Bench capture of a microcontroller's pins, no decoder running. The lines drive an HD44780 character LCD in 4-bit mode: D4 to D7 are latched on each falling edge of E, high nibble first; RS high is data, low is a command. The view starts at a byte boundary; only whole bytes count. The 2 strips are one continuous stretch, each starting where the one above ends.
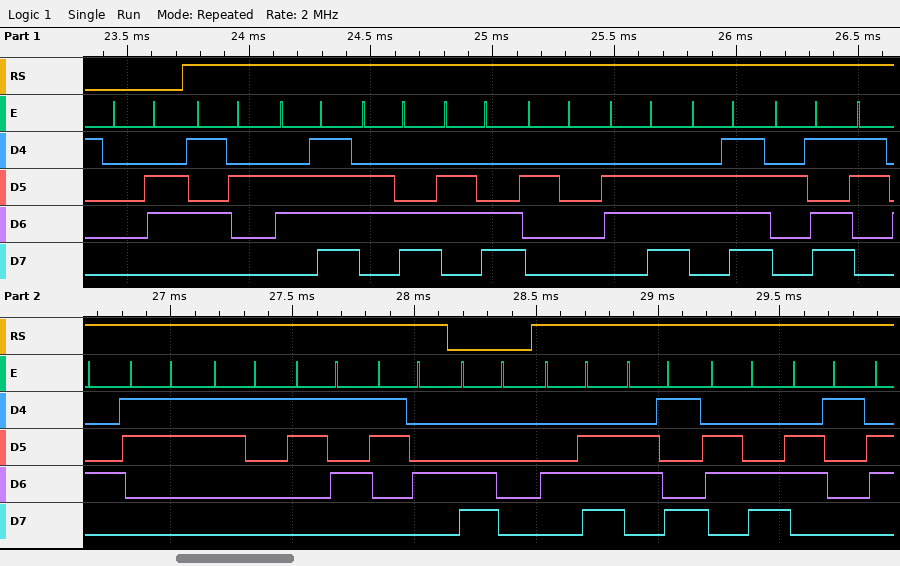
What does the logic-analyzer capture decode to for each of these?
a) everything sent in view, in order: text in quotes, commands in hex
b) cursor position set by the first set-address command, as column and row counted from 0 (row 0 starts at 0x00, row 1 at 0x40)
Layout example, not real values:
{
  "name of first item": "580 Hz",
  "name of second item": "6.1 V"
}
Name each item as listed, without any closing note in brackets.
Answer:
{
  "everything sent in view, in order: text in quotes, commands in hex": "0x06 \"Roll no-43154\" 0xC0 \"Nila\"",
  "cursor position set by the first set-address command, as column and row counted from 0": "column 0, row 1"
}
